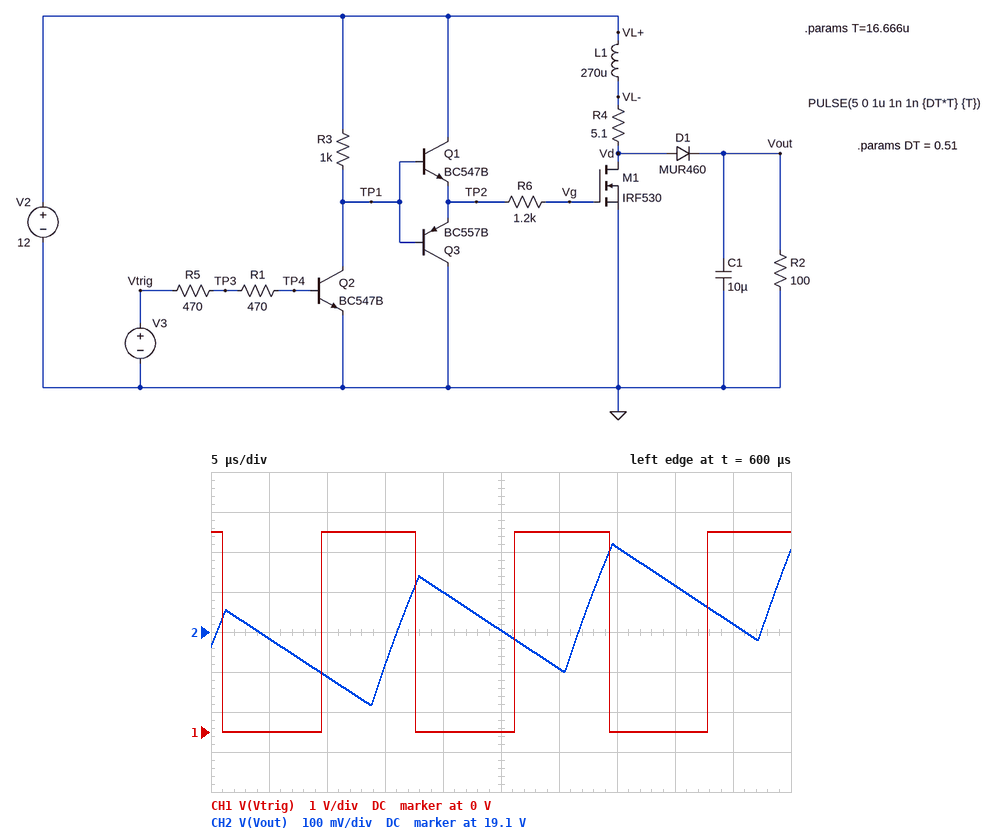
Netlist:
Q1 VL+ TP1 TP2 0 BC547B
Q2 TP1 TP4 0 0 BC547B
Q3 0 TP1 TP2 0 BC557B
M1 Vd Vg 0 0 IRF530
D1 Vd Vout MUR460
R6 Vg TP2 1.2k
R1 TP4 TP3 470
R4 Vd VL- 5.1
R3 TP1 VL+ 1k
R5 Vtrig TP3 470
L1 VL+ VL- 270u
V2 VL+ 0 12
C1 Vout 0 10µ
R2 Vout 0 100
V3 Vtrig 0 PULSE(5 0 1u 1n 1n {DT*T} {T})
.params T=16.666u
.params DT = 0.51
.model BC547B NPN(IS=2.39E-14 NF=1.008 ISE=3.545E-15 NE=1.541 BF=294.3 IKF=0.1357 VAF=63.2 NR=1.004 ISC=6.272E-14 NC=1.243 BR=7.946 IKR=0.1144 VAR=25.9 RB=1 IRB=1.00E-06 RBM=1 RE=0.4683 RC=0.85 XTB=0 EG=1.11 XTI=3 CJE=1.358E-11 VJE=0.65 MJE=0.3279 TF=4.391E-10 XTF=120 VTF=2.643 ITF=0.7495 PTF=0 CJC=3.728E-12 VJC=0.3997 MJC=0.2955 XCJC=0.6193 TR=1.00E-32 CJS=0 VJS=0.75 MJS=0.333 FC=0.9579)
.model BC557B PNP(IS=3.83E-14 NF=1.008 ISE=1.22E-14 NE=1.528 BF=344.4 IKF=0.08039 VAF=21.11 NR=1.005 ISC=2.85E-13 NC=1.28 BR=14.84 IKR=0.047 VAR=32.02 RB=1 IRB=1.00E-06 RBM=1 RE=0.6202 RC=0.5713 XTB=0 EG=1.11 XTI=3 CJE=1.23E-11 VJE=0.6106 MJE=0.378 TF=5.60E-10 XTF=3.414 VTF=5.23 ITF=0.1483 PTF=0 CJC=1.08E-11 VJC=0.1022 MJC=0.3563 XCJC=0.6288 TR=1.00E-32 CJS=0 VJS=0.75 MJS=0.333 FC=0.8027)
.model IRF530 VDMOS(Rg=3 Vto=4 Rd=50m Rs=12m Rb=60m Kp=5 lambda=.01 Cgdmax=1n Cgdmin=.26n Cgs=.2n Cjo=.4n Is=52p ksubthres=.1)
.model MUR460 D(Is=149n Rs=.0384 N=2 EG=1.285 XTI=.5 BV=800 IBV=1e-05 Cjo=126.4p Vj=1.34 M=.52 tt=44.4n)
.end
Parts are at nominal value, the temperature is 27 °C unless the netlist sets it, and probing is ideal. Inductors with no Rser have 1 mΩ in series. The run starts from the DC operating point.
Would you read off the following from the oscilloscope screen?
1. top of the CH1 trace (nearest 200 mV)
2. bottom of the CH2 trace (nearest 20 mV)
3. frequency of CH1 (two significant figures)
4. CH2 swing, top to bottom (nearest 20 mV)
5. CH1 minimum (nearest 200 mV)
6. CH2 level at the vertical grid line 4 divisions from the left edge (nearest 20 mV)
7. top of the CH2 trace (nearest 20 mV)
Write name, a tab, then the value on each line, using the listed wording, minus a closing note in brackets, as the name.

top of the CH1 trace	5.0 V
bottom of the CH2 trace	18.92 V
frequency of CH1	60 kHz
CH2 swing, top to bottom	400 mV
CH1 minimum	0 V
CH2 level at the vertical grid line 4 divisions from the left edge	19.20 V
top of the CH2 trace	19.32 V
